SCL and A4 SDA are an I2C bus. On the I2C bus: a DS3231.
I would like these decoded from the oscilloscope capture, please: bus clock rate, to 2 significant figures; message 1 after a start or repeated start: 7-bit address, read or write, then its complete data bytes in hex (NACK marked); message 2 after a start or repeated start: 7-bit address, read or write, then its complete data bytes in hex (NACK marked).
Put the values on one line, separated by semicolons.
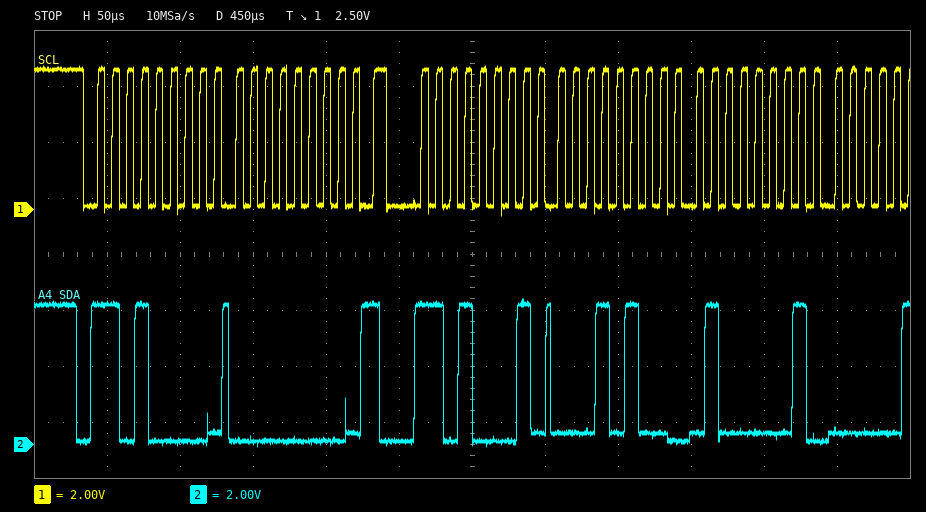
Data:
100 kHz; 0x68 write: 00; 0x68 read: 14 41
